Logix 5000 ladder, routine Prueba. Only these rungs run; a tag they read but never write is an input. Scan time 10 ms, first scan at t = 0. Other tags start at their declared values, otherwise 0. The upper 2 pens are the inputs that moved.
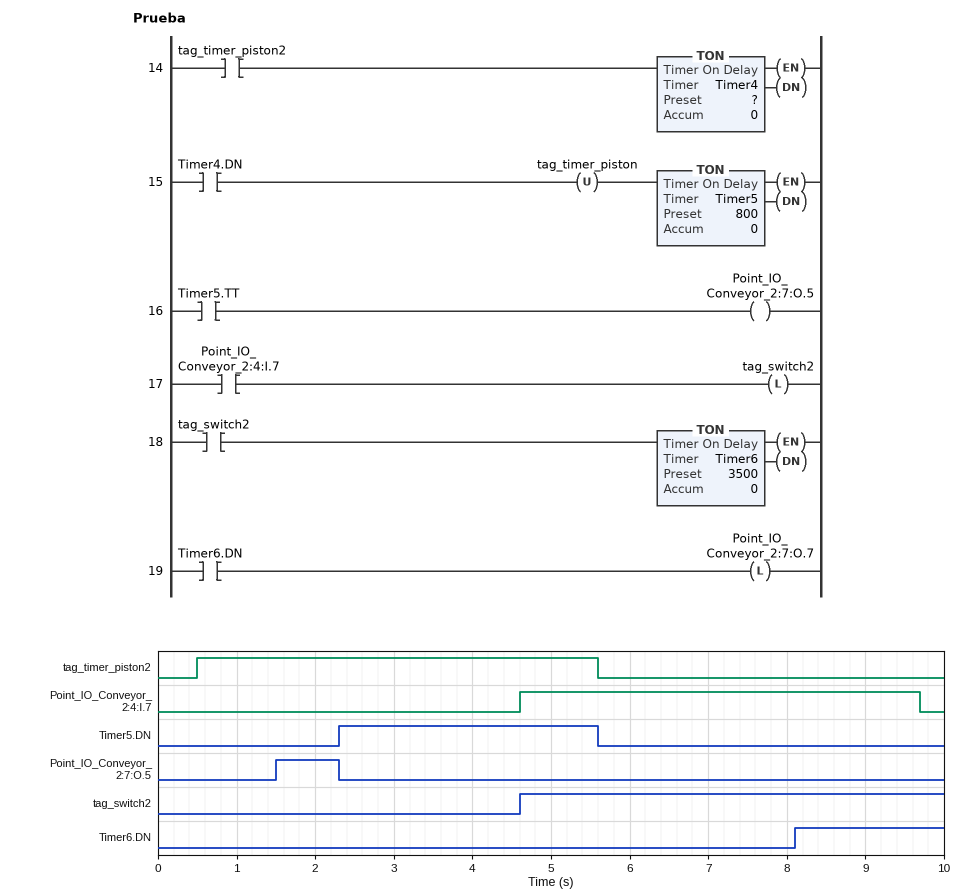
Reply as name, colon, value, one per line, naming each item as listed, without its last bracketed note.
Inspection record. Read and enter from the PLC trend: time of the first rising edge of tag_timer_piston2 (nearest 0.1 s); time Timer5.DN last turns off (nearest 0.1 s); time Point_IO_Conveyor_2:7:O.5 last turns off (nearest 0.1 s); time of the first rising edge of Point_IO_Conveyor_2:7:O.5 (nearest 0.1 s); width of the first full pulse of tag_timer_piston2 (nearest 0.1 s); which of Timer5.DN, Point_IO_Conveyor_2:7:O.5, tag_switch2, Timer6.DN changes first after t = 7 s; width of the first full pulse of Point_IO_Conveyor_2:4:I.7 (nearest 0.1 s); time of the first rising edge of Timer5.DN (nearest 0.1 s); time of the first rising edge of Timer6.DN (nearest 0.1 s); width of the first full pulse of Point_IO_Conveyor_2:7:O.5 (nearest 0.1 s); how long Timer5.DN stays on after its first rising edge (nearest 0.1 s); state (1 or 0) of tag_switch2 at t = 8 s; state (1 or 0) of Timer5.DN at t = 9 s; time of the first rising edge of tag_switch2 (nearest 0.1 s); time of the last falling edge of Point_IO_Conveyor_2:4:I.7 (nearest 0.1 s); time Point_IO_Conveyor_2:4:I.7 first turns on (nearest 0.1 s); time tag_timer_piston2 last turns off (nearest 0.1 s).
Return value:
time of the first rising edge of tag_timer_piston2: 0.5 s
time Timer5.DN last turns off: 5.6 s
time Point_IO_Conveyor_2:7:O.5 last turns off: 2.3 s
time of the first rising edge of Point_IO_Conveyor_2:7:O.5: 1.5 s
width of the first full pulse of tag_timer_piston2: 5.1 s
which of Timer5.DN, Point_IO_Conveyor_2:7:O.5, tag_switch2, Timer6.DN changes first after t = 7 s: Timer6.DN
width of the first full pulse of Point_IO_Conveyor_2:4:I.7: 5.1 s
time of the first rising edge of Timer5.DN: 2.3 s
time of the first rising edge of Timer6.DN: 8.1 s
width of the first full pulse of Point_IO_Conveyor_2:7:O.5: 0.8 s
how long Timer5.DN stays on after its first rising edge: 3.3 s
state (1 or 0) of tag_switch2 at t = 8 s: 1
state (1 or 0) of Timer5.DN at t = 9 s: 0
time of the first rising edge of tag_switch2: 4.6 s
time of the last falling edge of Point_IO_Conveyor_2:4:I.7: 9.7 s
time Point_IO_Conveyor_2:4:I.7 first turns on: 4.6 s
time tag_timer_piston2 last turns off: 5.6 s
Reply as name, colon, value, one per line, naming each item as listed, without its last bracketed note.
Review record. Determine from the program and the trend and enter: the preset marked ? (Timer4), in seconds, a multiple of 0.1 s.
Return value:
the preset marked ? (Timer4), in seconds, a multiple of 0.1 s: 1.0 s
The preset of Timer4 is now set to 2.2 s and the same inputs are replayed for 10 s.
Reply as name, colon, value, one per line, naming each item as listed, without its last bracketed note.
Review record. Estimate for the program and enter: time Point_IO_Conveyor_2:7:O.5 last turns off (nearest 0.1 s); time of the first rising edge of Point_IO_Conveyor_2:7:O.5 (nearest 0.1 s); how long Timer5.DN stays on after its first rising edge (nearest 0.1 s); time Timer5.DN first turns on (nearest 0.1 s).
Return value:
time Point_IO_Conveyor_2:7:O.5 last turns off: 3.5 s
time of the first rising edge of Point_IO_Conveyor_2:7:O.5: 2.7 s
how long Timer5.DN stays on after its first rising edge: 2.1 s
time Timer5.DN first turns on: 3.5 s
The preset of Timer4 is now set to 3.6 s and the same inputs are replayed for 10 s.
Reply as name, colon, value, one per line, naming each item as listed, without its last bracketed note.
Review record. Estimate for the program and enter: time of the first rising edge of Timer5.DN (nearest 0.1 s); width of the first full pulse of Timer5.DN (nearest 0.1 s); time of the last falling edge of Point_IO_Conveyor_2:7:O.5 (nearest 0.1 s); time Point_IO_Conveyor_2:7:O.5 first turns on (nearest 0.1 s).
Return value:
time of the first rising edge of Timer5.DN: 4.9 s
width of the first full pulse of Timer5.DN: 0.7 s
time of the last falling edge of Point_IO_Conveyor_2:7:O.5: 4.9 s
time Point_IO_Conveyor_2:7:O.5 first turns on: 4.1 s
